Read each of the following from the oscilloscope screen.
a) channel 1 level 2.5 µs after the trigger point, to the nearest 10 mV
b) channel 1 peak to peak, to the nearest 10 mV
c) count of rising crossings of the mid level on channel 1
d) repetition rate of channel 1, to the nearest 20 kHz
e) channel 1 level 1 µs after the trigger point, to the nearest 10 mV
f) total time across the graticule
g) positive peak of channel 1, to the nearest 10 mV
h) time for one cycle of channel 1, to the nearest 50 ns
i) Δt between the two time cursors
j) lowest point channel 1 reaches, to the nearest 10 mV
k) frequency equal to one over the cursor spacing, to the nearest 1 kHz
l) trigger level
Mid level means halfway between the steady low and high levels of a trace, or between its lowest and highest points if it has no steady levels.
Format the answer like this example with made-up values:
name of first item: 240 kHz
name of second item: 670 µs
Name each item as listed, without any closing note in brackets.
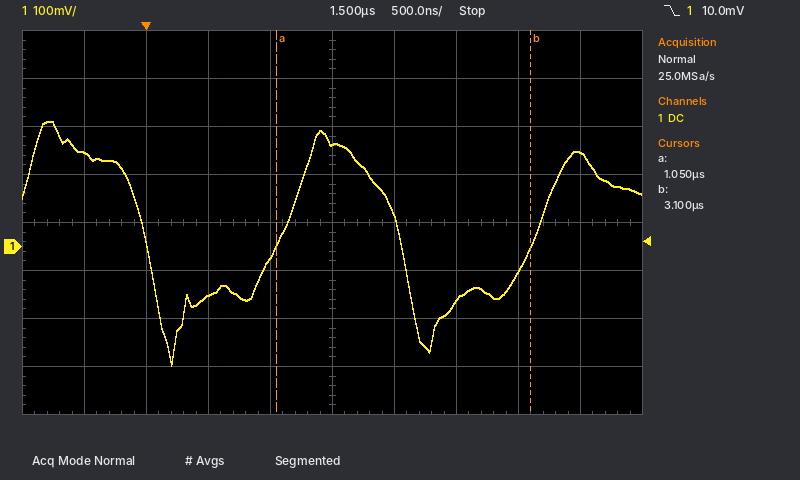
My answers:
channel 1 level 2.5 µs after the trigger point, to the nearest 10 mV: -110 mV
channel 1 peak to peak, to the nearest 10 mV: 510 mV
count of rising crossings of the mid level on channel 1: 2
repetition rate of channel 1, to the nearest 20 kHz: 480 kHz
channel 1 level 1 µs after the trigger point, to the nearest 10 mV: -20 mV
total time across the graticule: 5 µs
positive peak of channel 1, to the nearest 10 mV: 260 mV
time for one cycle of channel 1, to the nearest 50 ns: 2.05 µs
Δt between the two time cursors: 2.05 µs
lowest point channel 1 reaches, to the nearest 10 mV: -250 mV
frequency equal to one over the cursor spacing, to the nearest 1 kHz: 488 kHz
trigger level: 10.0 mV
